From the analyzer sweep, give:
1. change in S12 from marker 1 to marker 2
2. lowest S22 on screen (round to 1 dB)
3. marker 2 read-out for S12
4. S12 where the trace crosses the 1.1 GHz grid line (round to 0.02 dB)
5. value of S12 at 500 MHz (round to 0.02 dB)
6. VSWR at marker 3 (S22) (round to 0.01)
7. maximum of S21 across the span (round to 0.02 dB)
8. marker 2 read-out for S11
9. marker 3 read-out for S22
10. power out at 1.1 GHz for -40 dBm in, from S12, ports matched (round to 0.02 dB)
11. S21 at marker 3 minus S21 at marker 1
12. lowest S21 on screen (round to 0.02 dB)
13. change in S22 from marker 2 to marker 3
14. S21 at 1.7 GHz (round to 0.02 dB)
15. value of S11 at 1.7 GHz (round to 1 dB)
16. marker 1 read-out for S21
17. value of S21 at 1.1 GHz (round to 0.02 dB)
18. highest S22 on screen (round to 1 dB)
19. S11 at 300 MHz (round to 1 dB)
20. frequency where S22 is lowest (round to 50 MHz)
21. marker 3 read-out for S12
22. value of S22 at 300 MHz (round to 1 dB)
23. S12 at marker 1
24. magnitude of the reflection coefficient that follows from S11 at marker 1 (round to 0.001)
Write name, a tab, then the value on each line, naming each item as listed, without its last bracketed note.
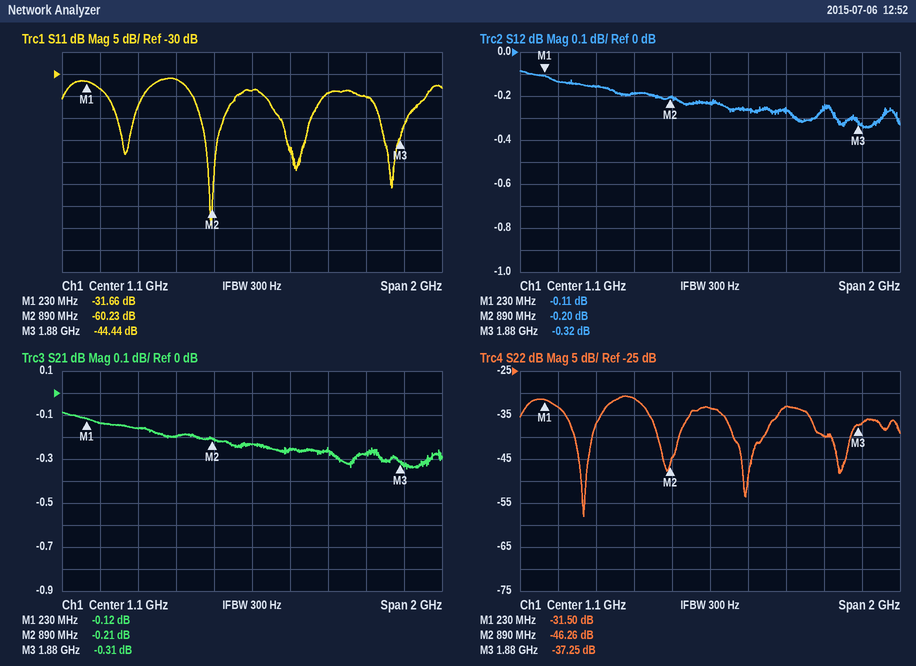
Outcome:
change in S12 from marker 1 to marker 2	-0.09 dB
lowest S22 on screen	-58 dB
marker 2 read-out for S12	-0.20 dB
S12 where the trace crosses the 1.1 GHz grid line	-0.24 dB
value of S12 at 500 MHz	-0.16 dB
VSWR at marker 3 (S22)	1.03
maximum of S21 across the span	-0.08 dB
marker 2 read-out for S11	-60.23 dB
marker 3 read-out for S22	-37.25 dB
power out at 1.1 GHz for -40 dBm in, from S12, ports matched	-40.24 dBm
S21 at marker 3 minus S21 at marker 1	-0.19 dB
lowest S21 on screen	-0.34 dB
change in S22 from marker 2 to marker 3	9.01 dB
S21 at 1.7 GHz	-0.28 dB
value of S11 at 1.7 GHz	-35 dB
marker 1 read-out for S21	-0.12 dB
value of S21 at 1.1 GHz	-0.24 dB
highest S22 on screen	-31 dB
S11 at 300 MHz	-33 dB
frequency where S22 is lowest	450 MHz
marker 3 read-out for S12	-0.32 dB
value of S22 at 300 MHz	-33 dB
S12 at marker 1	-0.11 dB
magnitude of the reflection coefficient that follows from S11 at marker 1	0.026
